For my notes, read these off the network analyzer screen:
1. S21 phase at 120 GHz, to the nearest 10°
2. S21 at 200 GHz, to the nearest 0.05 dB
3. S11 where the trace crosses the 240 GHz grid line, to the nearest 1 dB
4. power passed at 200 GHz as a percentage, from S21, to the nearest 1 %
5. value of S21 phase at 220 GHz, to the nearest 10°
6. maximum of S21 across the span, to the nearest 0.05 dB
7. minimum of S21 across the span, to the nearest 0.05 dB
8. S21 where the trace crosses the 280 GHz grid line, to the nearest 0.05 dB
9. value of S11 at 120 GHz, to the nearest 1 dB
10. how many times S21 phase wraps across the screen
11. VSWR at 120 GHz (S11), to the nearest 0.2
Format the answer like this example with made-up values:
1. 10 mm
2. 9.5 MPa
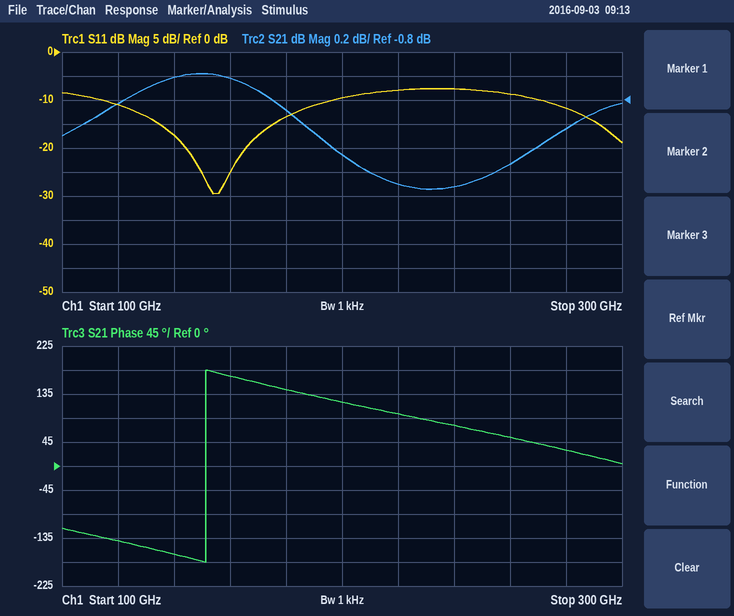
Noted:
1. -140°
2. -1.25 dB
3. -8 dB
4. 75 %
5. 100°
6. -0.60 dB
7. -1.55 dB
8. -1.05 dB
9. -11 dB
10. 1
11. 1.8
